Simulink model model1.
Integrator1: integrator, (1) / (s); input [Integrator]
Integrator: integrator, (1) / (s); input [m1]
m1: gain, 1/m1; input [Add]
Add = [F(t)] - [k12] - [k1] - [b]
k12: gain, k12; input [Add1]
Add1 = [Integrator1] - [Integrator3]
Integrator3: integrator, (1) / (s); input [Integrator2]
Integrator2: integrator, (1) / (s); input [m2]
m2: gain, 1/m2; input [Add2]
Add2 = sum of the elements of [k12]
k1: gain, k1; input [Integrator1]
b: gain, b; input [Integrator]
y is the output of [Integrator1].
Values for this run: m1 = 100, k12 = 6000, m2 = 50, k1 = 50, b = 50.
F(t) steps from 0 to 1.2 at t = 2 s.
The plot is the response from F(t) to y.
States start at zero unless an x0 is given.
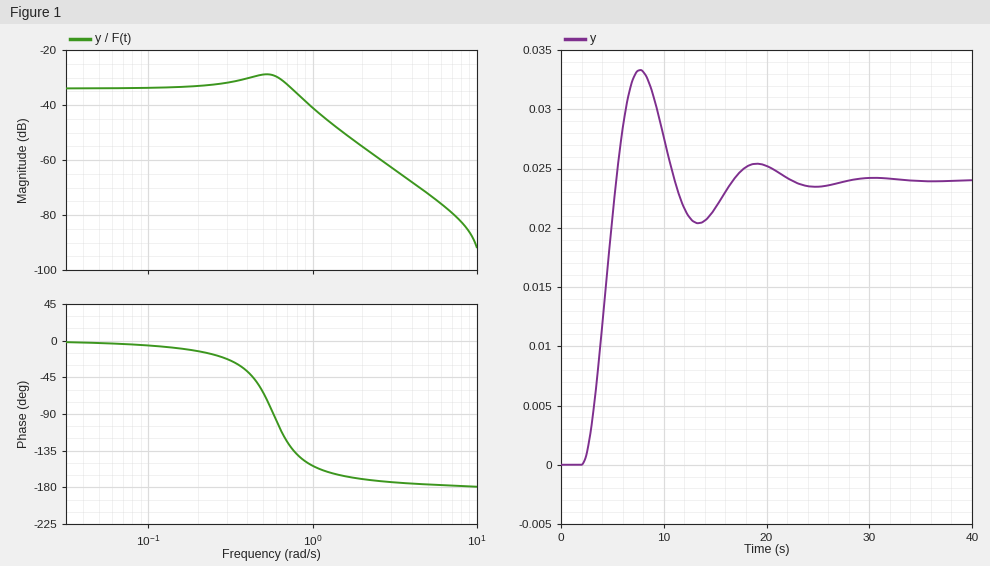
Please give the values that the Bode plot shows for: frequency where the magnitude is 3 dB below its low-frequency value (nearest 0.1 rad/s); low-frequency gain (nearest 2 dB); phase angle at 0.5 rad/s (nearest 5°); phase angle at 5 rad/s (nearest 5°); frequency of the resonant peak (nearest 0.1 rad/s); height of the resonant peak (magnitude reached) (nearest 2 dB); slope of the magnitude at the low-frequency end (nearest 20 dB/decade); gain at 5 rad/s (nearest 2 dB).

0.8 rad/s
-34 dB
-65°
-175°
0.5 rad/s
-28 dB
0 dB/decade
-72 dB
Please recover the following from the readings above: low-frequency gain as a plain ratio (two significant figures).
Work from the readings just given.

0.020
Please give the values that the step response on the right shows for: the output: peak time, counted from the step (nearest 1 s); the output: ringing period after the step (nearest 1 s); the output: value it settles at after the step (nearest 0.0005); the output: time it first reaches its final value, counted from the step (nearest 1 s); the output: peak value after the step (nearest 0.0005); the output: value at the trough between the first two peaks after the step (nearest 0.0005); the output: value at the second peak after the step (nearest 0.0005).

6 s
11 s
0.0240
3 s
0.0335
0.0205
0.0255
